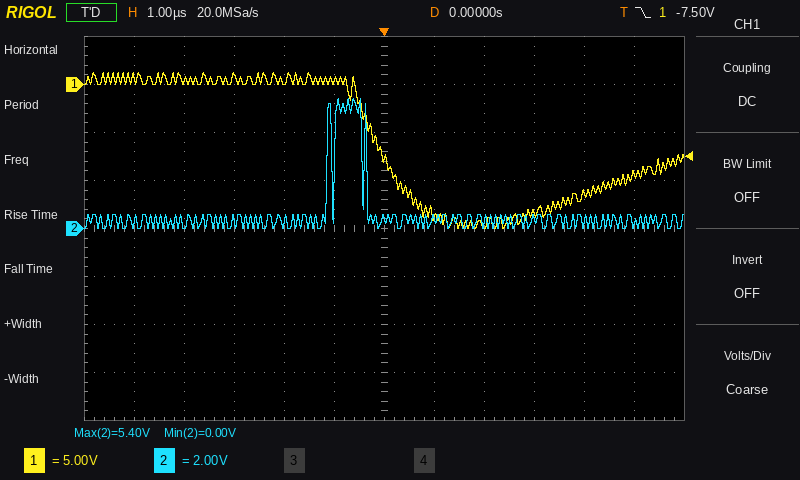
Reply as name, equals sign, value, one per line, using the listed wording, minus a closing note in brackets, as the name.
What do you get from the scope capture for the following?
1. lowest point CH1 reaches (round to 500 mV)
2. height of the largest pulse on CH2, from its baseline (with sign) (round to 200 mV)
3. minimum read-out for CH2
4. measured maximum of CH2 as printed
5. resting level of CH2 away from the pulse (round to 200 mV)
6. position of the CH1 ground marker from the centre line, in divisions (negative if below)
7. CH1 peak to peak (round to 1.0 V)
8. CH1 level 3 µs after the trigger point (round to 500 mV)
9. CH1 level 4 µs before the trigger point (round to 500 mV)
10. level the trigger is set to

lowest point CH1 reaches = -15.0 V
height of the largest pulse on CH2, from its baseline (with sign) = +5.0 V
minimum read-out for CH2 = 0.00 V
measured maximum of CH2 as printed = 5.40 V
resting level of CH2 away from the pulse = 400 mV
position of the CH1 ground marker from the centre line, in divisions = +3.0 div
CH1 peak to peak = 16.0 V
CH1 level 3 µs after the trigger point = -13.5 V
CH1 level 4 µs before the trigger point = 500 mV
level the trigger is set to = -7.50 V
